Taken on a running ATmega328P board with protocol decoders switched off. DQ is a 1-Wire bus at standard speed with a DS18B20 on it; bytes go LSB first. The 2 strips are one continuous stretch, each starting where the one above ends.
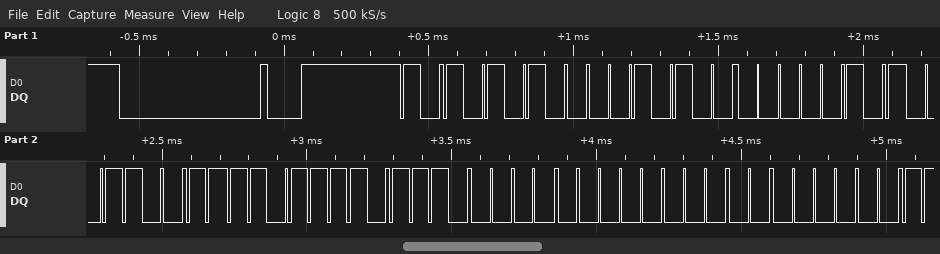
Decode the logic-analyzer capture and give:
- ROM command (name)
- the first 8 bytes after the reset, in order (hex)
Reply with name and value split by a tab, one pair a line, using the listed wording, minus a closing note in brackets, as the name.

ROM command	Match ROM
the first 8 bytes after the reset, in order	55 28 A0 CC 7B 07 00 00
